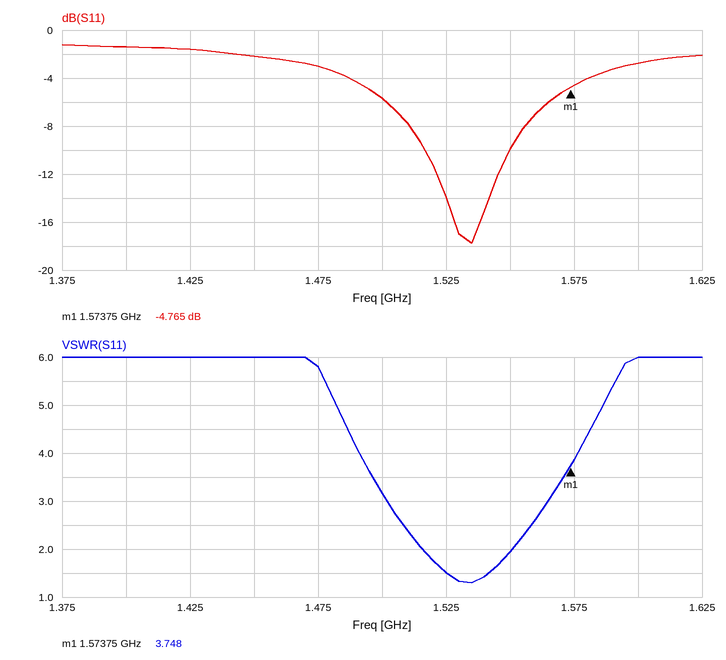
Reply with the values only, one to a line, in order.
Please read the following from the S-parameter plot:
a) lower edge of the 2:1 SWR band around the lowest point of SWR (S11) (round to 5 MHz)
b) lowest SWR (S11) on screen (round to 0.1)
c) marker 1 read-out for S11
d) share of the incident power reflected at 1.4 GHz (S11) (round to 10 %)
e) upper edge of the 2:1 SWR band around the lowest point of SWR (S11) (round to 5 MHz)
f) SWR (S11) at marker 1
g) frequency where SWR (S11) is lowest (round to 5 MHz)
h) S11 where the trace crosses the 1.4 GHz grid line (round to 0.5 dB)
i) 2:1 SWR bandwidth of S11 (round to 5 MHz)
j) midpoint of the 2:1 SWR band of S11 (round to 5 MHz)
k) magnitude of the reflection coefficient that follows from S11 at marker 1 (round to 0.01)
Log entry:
1.515 GHz
1.3
-4.765 dB
70 %
1.550 GHz
3.748
1.535 GHz
-1.5 dB
35 MHz
1.535 GHz
0.58
